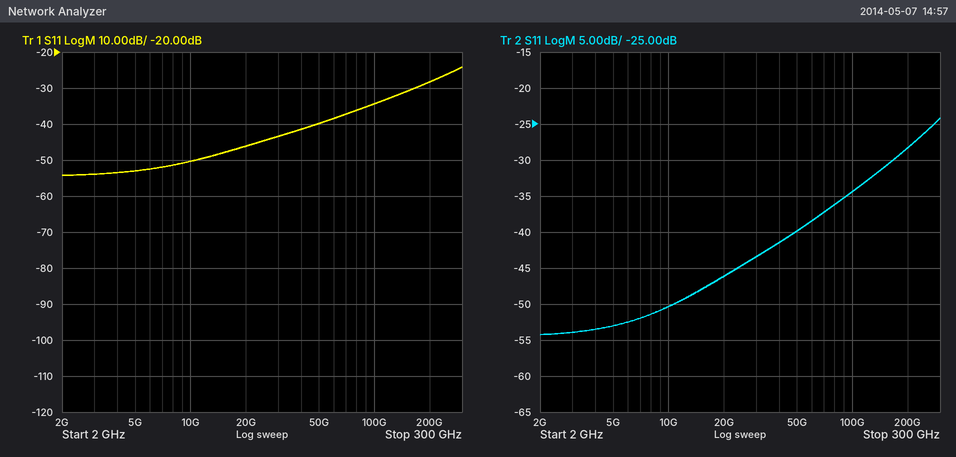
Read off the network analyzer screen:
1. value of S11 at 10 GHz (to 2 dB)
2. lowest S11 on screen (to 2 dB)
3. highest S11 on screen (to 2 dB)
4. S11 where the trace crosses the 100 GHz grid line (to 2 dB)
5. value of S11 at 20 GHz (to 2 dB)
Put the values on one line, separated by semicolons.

-50 dB; -54 dB; -24 dB; -34 dB; -46 dB
